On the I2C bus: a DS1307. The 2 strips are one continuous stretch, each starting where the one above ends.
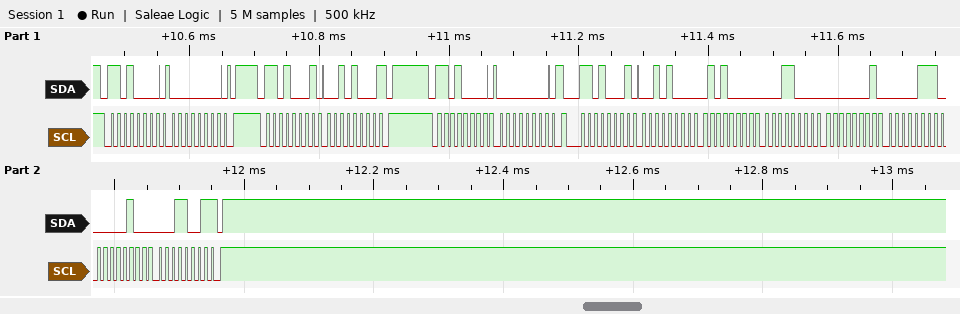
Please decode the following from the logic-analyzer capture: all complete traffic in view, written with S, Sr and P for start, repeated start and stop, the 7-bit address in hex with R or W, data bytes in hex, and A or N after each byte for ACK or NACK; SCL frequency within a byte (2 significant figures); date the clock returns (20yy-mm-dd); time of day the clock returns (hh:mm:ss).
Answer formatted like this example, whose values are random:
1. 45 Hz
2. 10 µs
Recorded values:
1. S 68W A 00 A P S 68R A 28 N P S 68W A 00 A Sr 68R A 28 A 50 A 18 A 01 A 07 A 04 A 19 N P
2. 100 kHz
3. 2019-04-07
4. 18:50:28
